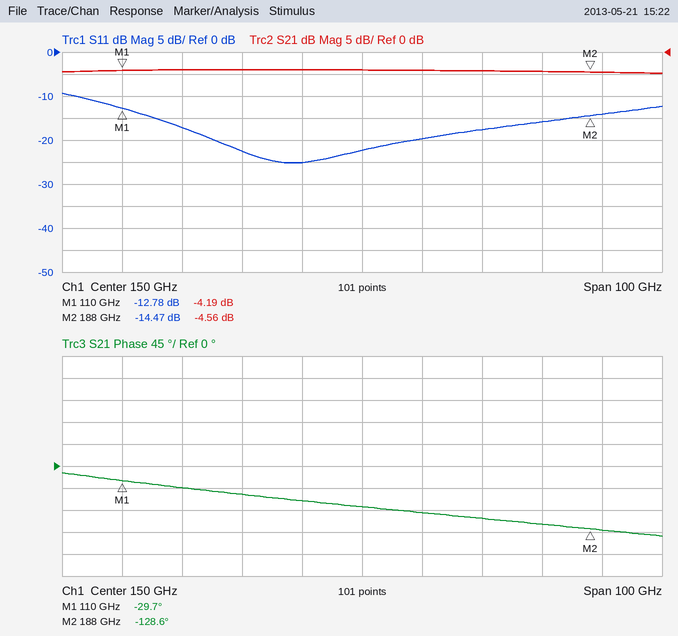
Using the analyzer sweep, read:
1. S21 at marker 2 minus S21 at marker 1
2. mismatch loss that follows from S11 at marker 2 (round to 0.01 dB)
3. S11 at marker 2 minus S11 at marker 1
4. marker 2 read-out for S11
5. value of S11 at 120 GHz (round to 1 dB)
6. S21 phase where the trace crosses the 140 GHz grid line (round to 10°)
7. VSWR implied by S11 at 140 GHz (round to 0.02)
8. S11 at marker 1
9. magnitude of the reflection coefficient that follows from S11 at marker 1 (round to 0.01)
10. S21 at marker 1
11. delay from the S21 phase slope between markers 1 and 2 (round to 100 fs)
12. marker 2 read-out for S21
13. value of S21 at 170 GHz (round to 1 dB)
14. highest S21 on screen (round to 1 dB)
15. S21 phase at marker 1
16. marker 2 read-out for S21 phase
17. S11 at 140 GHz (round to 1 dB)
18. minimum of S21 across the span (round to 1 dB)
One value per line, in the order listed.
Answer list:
-0.37 dB
0.16 dB
-1.69 dB
-14.47 dB
-17 dB
-70°
1.12
-12.78 dB
0.23
-4.19 dB
3.5 ps
-4.56 dB
-4 dB
-4 dB
-29.7°
-128.6°
-25 dB
-5 dB
